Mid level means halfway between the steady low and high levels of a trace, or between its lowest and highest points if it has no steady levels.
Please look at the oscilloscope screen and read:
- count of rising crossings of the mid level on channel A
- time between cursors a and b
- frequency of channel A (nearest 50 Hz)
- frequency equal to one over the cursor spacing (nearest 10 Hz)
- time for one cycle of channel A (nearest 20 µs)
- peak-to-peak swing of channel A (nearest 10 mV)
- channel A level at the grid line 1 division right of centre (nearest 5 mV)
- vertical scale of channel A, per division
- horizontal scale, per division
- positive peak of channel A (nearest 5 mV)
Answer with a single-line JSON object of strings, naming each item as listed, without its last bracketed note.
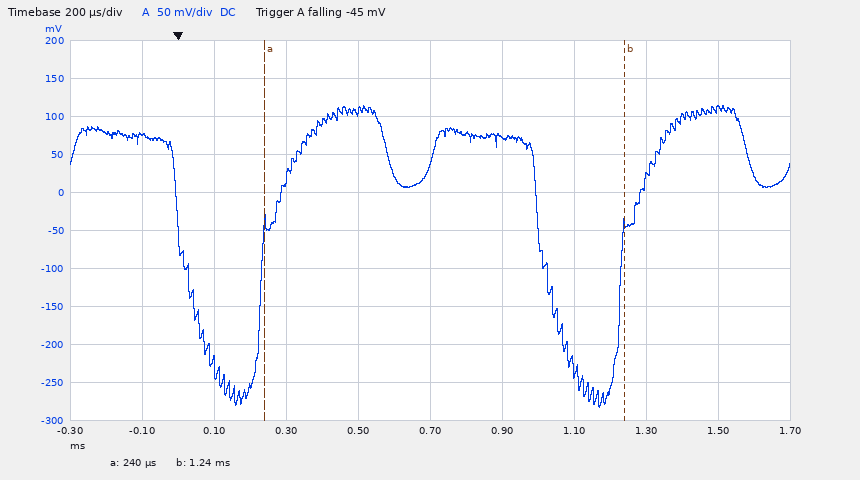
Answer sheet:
{"count of rising crossings of the mid level on channel A": "2", "time between cursors a and b": "1.00 ms", "frequency of channel A": "1.00 kHz", "frequency equal to one over the cursor spacing": "1.00 kHz", "time for one cycle of channel A": "1.00 ms", "peak-to-peak swing of channel A": "400 mV", "channel A level at the grid line 1 division right of centre": "70 mV", "vertical scale of channel A, per division": "50 mV", "horizontal scale, per division": "200 µs", "positive peak of channel A": "115 mV"}
